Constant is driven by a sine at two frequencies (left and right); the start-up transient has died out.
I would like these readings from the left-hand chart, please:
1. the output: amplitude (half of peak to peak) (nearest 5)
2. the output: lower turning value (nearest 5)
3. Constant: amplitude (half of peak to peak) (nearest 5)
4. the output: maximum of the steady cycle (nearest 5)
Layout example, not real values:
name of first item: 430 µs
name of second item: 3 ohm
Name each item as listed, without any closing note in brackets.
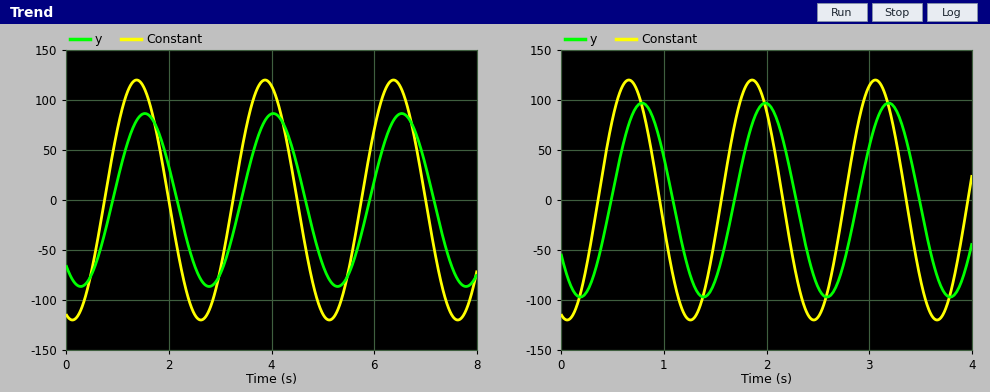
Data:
the output: amplitude (half of peak to peak): 85
the output: lower turning value: -85
Constant: amplitude (half of peak to peak): 120
the output: maximum of the steady cycle: 85
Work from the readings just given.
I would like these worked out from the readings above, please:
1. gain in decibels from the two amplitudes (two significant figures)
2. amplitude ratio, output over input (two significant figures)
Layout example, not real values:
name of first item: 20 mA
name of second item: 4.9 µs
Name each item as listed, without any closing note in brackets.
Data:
gain in decibels from the two amplitudes: -3.0 dB
amplitude ratio, output over input: 0.71
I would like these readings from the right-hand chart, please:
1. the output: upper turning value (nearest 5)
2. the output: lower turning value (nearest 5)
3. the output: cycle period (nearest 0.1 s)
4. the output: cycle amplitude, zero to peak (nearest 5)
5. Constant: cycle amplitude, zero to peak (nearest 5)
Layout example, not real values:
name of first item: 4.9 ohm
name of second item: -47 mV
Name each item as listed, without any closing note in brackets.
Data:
the output: upper turning value: 95
the output: lower turning value: -95
the output: cycle period: 1.2 s
the output: cycle amplitude, zero to peak: 95
Constant: cycle amplitude, zero to peak: 120
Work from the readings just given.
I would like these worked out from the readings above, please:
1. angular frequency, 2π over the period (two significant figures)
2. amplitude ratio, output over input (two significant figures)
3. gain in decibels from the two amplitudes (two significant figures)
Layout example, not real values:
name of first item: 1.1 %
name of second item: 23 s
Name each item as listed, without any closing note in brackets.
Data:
angular frequency, 2π over the period: 5.2 rad/s
amplitude ratio, output over input: 0.79
gain in decibels from the two amplitudes: -2.0 dB
